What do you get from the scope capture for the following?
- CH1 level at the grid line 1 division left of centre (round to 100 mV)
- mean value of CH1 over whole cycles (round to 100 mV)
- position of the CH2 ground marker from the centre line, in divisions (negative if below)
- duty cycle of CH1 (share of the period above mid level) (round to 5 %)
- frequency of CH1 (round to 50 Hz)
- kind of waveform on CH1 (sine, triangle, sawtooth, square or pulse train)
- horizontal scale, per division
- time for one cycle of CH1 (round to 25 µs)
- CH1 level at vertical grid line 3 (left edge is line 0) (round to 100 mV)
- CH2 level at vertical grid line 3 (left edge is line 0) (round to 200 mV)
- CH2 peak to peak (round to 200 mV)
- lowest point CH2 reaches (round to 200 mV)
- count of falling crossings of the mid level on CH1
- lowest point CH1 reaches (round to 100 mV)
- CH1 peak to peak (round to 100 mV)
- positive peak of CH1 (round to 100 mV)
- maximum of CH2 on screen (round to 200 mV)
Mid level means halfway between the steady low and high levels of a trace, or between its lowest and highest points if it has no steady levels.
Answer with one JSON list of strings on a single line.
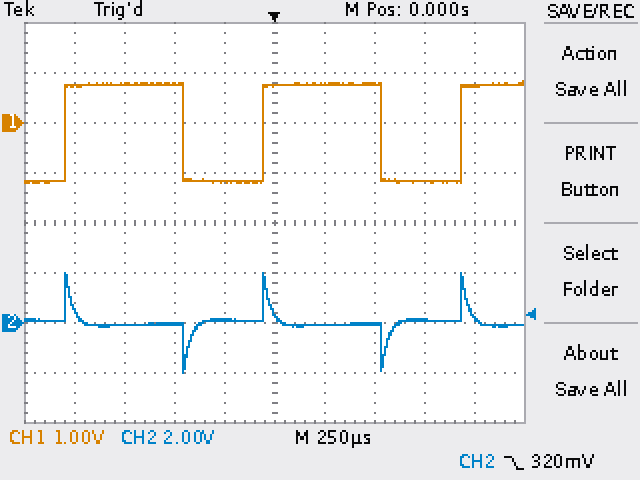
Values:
["-1.2 V", "0.0 V", "-2.0 div", "60 %", "1.00 kHz", "pulse train", "250 µs", "1.000 ms", "800 mV", "0.0 V", "4.0 V", "-2.0 V", "2", "-1.2 V", "2.0 V", "800 mV", "2.0 V"]
